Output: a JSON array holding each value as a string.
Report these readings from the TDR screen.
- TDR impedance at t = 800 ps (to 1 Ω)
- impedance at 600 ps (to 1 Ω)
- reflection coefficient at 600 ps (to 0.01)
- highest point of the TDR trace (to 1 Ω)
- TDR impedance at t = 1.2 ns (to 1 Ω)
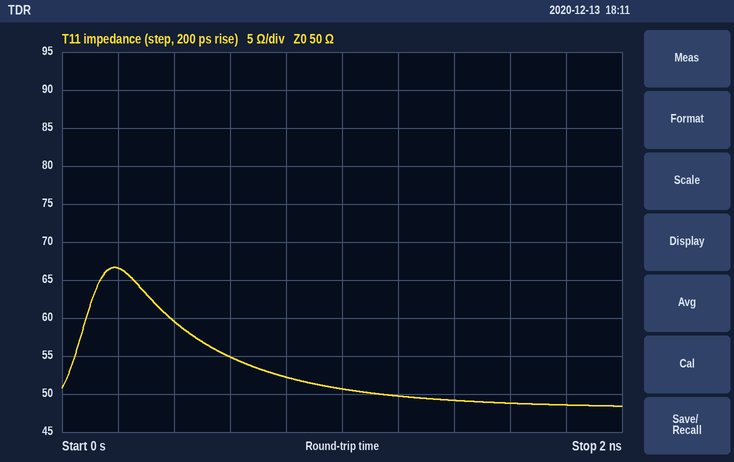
["52 Ω", "55 Ω", "+0.05", "67 Ω", "50 Ω"]
